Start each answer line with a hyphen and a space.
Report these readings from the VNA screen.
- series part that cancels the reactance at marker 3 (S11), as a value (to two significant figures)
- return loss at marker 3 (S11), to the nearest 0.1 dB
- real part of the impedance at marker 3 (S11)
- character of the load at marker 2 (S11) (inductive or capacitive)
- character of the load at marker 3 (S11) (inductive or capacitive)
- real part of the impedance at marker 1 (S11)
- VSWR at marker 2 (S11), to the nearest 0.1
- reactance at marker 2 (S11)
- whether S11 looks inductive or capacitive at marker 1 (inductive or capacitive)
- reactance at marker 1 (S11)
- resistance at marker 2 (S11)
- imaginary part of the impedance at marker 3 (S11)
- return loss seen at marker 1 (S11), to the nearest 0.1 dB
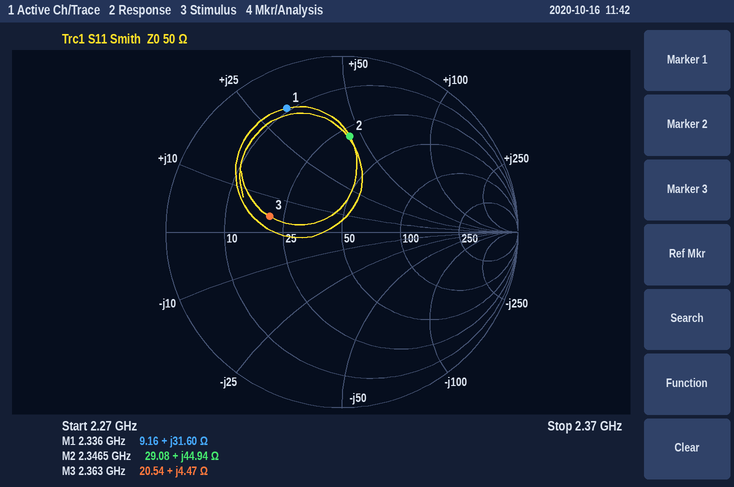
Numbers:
- 15 pF
- 7.5 dB
- 20.54 Ω
- inductive
- inductive
- 9.16 Ω
- 3.4
- +44.94 Ω
- inductive
- +31.60 Ω
- 29.08 Ω
- +4.47 Ω
- 2.3 dB
